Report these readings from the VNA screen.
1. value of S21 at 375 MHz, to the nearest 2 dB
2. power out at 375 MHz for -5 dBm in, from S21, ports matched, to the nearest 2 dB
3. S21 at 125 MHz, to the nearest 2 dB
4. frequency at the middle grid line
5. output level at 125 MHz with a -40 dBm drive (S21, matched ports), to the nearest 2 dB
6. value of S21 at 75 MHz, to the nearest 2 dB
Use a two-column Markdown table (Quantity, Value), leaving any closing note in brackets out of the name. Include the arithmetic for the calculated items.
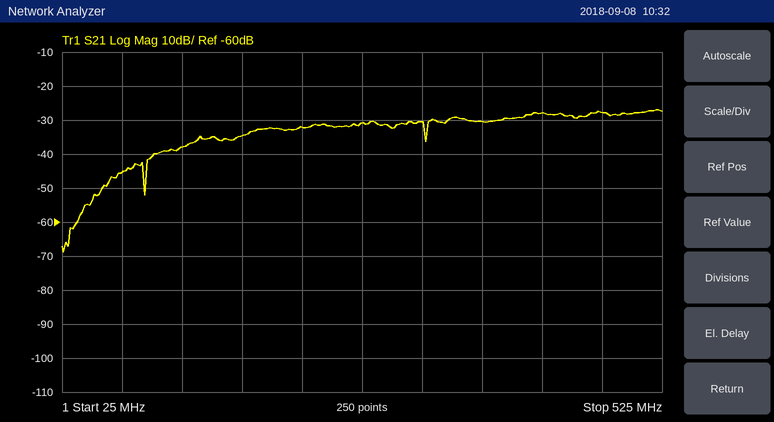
| Quantity | Value |
|---|---|
| value of S21 at 375 MHz, to the nearest 2 dB | -30 dB |
| power out at 375 MHz for -5 dBm in, from S21, ports matched, to the nearest 2 dB | -5 dBm + (-30 dB) = -36 dBm |
| S21 at 125 MHz, to the nearest 2 dB | -38 dB |
| frequency at the middle grid line | 275 MHz |
| output level at 125 MHz with a -40 dBm drive (S21, matched ports), to the nearest 2 dB | -40 dBm + (-38 dB) = -78 dBm |
| value of S21 at 75 MHz, to the nearest 2 dB | -46 dB |
